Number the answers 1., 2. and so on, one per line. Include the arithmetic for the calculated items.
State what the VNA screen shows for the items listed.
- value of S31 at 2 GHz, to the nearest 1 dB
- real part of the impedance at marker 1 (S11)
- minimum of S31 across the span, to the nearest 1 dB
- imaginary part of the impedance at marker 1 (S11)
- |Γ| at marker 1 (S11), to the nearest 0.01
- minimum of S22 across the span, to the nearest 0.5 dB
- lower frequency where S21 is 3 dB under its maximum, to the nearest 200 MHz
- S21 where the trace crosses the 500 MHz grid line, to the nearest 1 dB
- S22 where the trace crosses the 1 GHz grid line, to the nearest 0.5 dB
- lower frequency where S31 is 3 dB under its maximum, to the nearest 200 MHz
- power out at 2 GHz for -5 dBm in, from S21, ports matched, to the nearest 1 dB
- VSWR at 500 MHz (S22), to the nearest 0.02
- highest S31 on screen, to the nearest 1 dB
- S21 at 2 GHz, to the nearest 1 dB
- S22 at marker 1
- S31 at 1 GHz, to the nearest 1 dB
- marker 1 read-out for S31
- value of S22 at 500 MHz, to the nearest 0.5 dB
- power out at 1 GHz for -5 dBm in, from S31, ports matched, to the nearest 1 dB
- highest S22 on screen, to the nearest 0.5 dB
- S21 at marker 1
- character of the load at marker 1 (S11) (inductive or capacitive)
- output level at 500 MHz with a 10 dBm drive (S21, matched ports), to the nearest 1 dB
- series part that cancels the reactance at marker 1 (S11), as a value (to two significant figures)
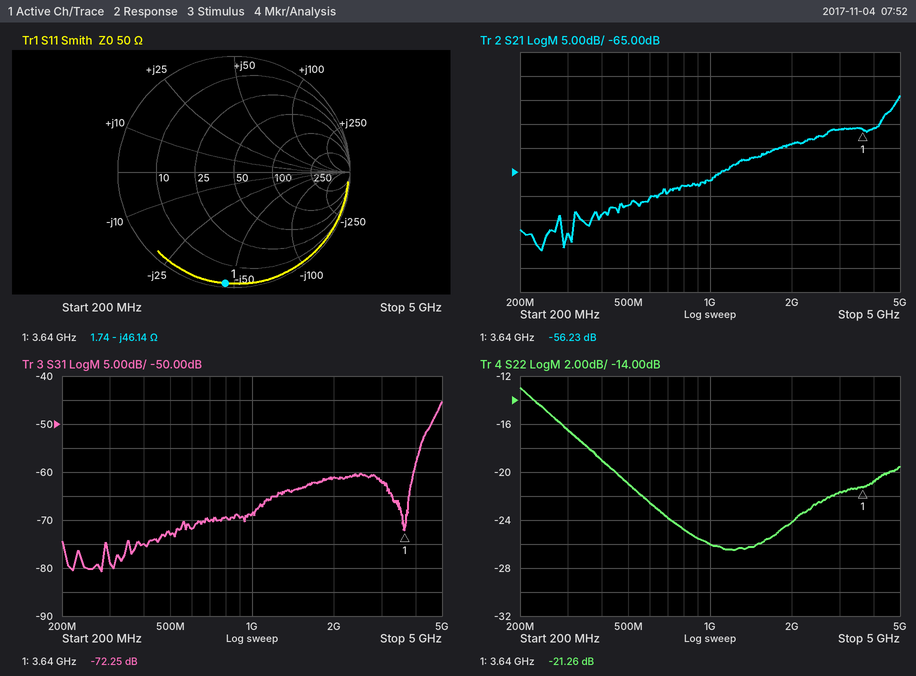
1. -61 dB
2. 1.74 Ω
3. -81 dB
4. -46.14 Ω
5. 0.96
6. -26.5 dB
7. 4.6 GHz
8. -72 dB
9. -26.0 dB
10. 4.8 GHz
11. -5 dBm + (-59 dB) = -64 dBm
12. |Γ| = 10^(-21/20) = 0.0891; VSWR = (1 + 0.0891)/(1 − 0.0891) ≈ 1.20
13. -45 dB
14. -59 dB
15. -21.26 dB
16. -69 dB
17. -72.25 dB
18. -21.0 dB
19. -5 dBm + (-69 dB) = -74 dBm
20. -13.0 dB
21. -56.23 dB
22. capacitive
23. 10 dBm + (-72 dB) = -62 dBm
24. L = 46.14 Ω/(2π × 3.64 GHz) ≈ 2.0 nH
